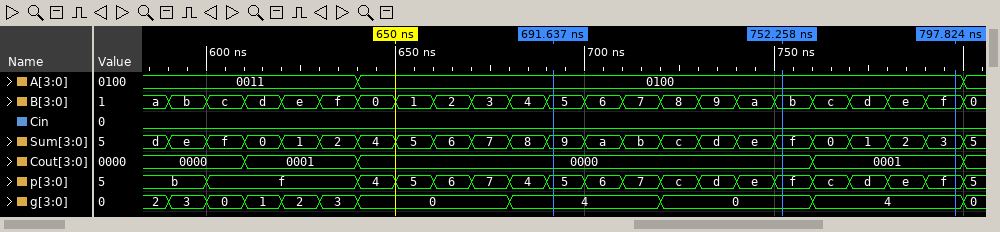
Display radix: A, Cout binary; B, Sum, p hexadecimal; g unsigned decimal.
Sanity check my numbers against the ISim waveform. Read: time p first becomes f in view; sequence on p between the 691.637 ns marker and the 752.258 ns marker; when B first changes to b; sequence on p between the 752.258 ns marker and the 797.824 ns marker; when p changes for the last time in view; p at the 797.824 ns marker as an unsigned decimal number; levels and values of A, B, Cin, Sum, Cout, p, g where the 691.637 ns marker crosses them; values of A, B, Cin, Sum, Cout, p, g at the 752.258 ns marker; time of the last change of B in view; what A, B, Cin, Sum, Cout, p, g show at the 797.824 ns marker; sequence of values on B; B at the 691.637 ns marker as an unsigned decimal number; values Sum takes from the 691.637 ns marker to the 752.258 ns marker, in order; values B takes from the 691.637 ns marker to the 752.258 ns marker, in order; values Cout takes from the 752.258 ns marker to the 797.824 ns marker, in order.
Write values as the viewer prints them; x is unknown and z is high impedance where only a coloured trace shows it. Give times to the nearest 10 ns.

600 ns
5, 6, 7, c, d, e, f
590 ns
f, c, d, e, f
800 ns
15
A=0100, B=5, Cin=0, Sum=9, Cout=0000, p=5, g=4
A=0100, B=b, Cin=0, Sum=f, Cout=0000, p=f, g=0
800 ns
A=0100, B=f, Cin=0, Sum=3, Cout=0001, p=f, g=4
a, b, c, d, e, f, 0, 1, 2, 3, 4, 5, 6, 7, 8, 9, a, b, c, d, e, f, 0
5
9, a, b, c, d, e, f
5, 6, 7, 8, 9, a, b
0000, 0001
